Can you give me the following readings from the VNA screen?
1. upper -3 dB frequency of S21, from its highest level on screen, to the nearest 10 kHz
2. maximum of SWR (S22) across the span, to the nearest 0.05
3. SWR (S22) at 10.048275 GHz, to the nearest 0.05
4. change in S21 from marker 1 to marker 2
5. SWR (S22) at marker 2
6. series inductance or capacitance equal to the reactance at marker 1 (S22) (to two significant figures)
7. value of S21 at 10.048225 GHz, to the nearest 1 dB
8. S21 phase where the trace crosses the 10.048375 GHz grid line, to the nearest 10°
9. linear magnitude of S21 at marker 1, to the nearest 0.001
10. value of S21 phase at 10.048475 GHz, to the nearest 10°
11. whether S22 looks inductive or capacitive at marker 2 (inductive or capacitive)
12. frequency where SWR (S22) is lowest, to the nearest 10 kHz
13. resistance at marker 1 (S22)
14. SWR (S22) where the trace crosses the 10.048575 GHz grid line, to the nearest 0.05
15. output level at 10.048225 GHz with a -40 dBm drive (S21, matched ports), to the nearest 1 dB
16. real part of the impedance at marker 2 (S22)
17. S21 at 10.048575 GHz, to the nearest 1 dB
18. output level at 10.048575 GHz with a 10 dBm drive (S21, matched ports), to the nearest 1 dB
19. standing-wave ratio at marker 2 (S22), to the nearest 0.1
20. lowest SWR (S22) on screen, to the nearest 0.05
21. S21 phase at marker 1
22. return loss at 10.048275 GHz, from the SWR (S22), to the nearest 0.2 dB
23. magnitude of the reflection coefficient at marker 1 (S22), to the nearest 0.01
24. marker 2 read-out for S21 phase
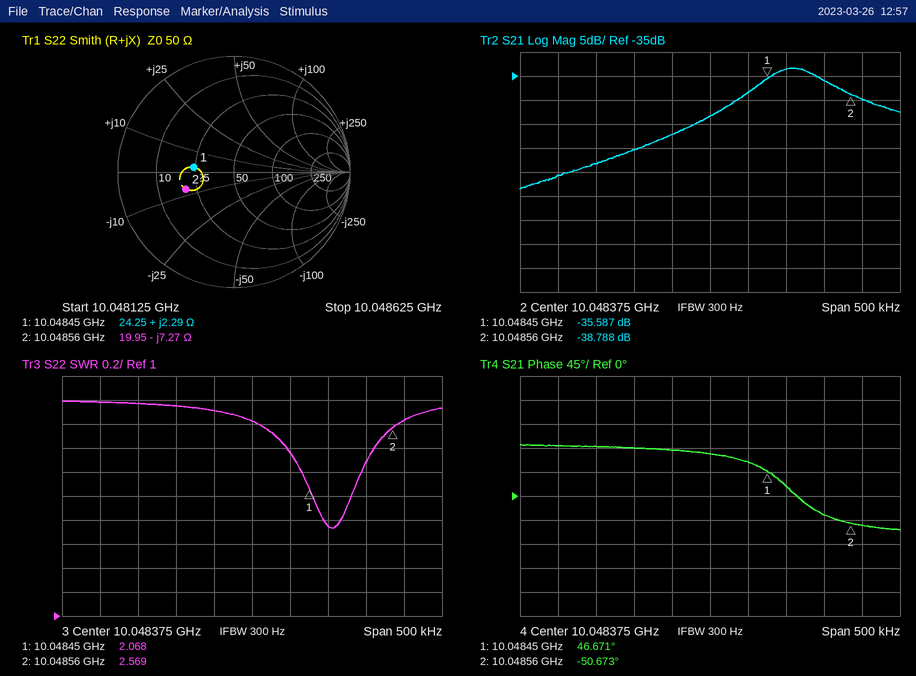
10.04853 GHz
2.80
2.75
-3.201 dB
2.569
36 pH
-53 dB
80°
0.017
20°
capacitive
10.04848 GHz
24.25 Ω
2.65
-93 dBm
19.95 Ω
-40 dB
-30 dBm
2.6
1.75
46.671°
6.6 dB
0.35
-50.673°
